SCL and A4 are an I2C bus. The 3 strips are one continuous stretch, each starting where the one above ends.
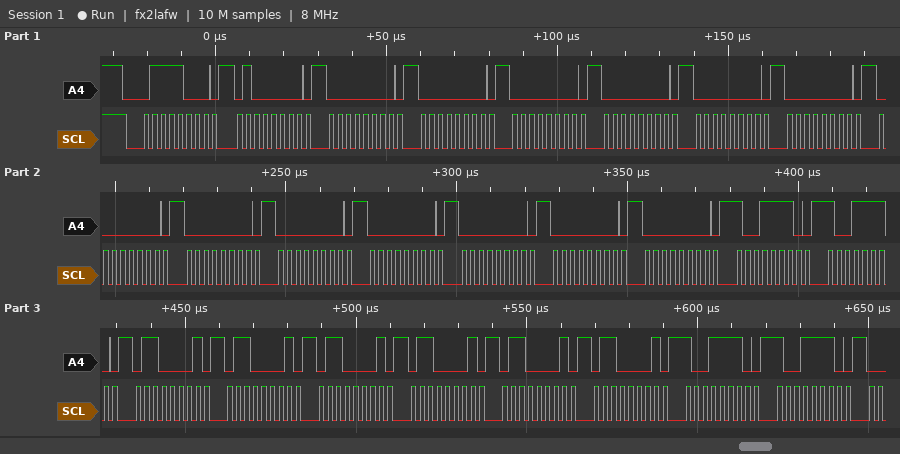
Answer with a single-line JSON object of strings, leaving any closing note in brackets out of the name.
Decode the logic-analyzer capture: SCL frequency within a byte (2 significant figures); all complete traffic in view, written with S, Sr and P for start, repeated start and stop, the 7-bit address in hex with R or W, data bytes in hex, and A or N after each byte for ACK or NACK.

{"SCL frequency within a byte": "400 kHz", "all complete traffic in view, written with S, Sr and P for start, repeated start and stop, the 7-bit address in hex with R or W, data bytes in hex, and A or N after each byte for ACK or NACK": "S 3CW A 40 A 00 A 00 A 00 A 00 A 00 A 00 A 00 A 00 A 00 A 00 A 00 A 00 A 00 A 9E A 9E A 61 A 61 A 61 A 61 A 61 A 61 A 9E A 9E A"}
